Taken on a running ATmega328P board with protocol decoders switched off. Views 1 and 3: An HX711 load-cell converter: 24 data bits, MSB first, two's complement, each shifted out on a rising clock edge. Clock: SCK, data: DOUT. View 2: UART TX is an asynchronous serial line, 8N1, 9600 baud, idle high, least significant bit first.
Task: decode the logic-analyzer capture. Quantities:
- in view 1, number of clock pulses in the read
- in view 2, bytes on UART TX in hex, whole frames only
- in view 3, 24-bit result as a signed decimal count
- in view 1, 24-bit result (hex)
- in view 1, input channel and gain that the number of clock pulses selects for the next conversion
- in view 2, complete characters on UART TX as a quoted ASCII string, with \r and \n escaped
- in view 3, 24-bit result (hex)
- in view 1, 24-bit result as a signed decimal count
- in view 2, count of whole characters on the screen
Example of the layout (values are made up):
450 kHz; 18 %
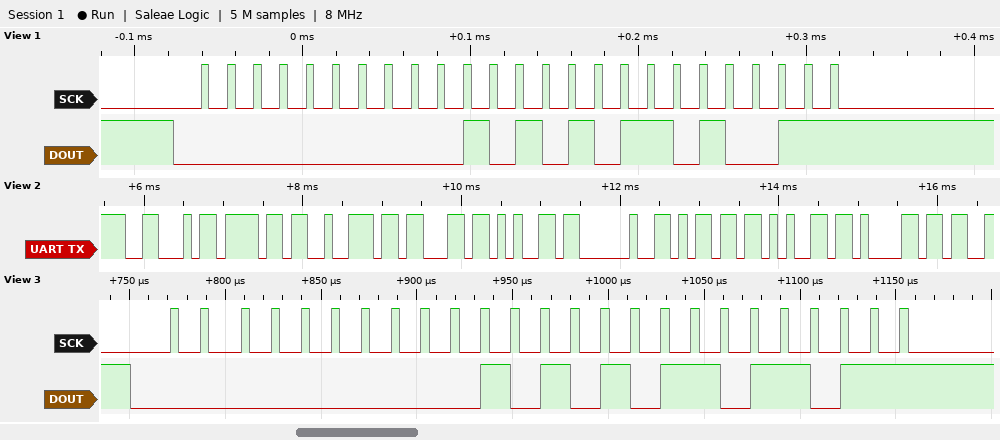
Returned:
25; 46 6F 72 63 65 20 6D 65 61; 10971; 0x002AD3; channel A, gain 128; "Force mea"; 0x002ADB; 10963; 9
